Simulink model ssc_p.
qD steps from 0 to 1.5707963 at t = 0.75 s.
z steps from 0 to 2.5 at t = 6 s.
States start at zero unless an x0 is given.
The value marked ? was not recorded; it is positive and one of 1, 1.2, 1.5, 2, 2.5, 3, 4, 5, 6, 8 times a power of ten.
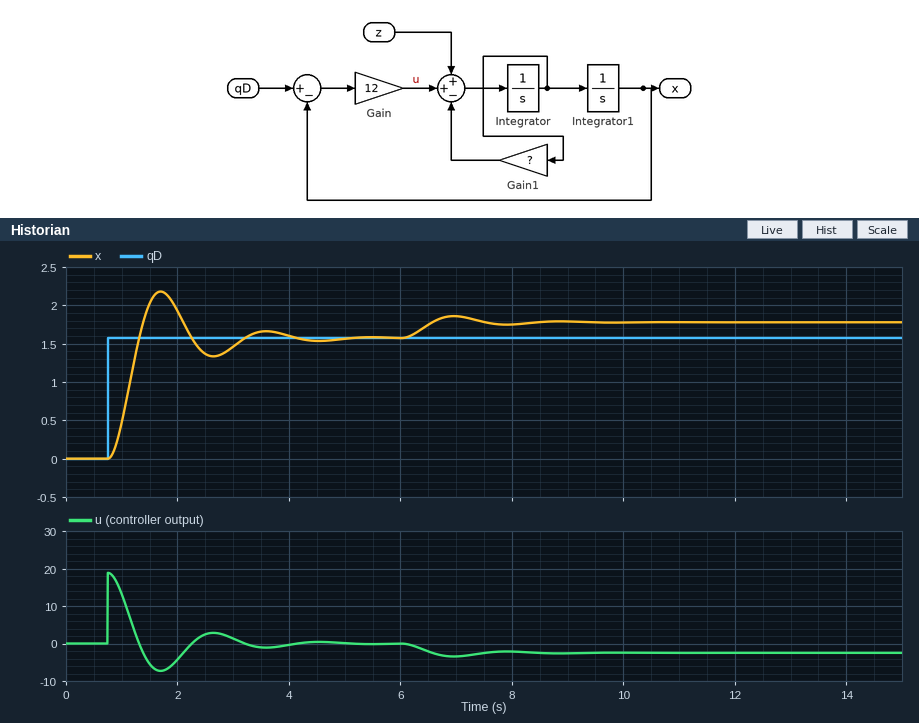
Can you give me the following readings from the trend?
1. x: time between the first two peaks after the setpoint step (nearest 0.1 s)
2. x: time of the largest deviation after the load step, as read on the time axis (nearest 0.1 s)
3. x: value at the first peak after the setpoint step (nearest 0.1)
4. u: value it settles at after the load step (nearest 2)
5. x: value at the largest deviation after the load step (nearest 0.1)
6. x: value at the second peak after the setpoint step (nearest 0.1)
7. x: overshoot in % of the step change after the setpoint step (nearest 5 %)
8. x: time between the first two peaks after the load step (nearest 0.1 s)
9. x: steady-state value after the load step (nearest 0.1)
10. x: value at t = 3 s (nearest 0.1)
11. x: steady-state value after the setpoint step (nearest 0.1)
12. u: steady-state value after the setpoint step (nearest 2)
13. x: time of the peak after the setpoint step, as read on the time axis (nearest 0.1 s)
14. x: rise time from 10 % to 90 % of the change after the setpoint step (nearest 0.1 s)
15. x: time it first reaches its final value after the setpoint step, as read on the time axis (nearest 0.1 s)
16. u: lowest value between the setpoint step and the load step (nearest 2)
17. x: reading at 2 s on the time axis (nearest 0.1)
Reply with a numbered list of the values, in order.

1. 1.9 s
2. 7.0 s
3. 2.2
4. -2
5. 1.9
6. 1.7
7. 40 %
8. 1.9 s
9. 1.8
10. 1.5
11. 1.6
12. 0
13. 1.7 s
14. 0.4 s
15. 1.3 s
16. -8
17. 1.9
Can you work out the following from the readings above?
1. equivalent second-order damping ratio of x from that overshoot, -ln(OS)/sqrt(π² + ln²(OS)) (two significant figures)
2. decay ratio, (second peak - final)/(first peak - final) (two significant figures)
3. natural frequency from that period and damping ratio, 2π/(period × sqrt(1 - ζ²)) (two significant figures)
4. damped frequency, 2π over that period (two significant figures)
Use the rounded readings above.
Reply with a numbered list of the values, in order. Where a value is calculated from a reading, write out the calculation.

1. ln(0.4) = -0.916; 0.916 / sqrt(9.870 + 0.840) = 0.28
2. (1.7 - 1.6) / (2.2 - 1.6) = 0.17
3. 2π / (1.9 × sqrt(1 - 0.28²)) = 3.4 rad/s
4. 2π / 1.9 = 3.3 rad/s
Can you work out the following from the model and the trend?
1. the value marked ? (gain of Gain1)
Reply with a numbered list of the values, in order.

1. 2
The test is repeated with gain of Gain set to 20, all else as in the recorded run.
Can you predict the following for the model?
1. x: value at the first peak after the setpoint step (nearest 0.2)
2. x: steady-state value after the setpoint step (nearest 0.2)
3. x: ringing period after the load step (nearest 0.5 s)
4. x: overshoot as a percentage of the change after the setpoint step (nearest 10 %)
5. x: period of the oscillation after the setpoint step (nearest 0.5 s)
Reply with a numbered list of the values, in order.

1. 2.4
2. 1.6
3. 1.5 s
4. 50 %
5. 1.5 s
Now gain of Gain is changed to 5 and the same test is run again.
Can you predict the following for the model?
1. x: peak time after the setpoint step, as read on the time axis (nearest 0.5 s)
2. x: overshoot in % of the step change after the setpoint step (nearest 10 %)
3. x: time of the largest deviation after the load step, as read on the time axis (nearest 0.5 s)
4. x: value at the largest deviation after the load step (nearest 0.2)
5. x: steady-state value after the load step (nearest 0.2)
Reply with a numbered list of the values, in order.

1. 2.5 s
2. 20 %
3. 7.5 s
4. 2.2
5. 2.0
